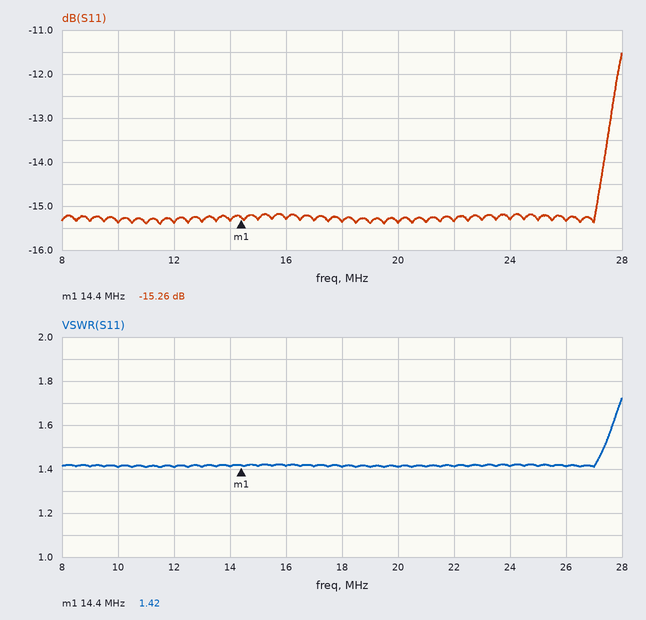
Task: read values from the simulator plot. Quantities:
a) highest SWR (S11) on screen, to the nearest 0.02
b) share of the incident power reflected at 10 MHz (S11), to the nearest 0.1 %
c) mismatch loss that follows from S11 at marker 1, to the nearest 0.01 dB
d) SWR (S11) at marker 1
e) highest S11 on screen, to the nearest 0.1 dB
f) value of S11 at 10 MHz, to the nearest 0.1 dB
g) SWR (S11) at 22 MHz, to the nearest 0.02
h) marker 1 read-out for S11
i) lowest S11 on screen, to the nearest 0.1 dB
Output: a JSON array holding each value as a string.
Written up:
["1.72", "2.9 %", "0.13 dB", "1.42", "-11.5 dB", "-15.4 dB", "1.42", "-15.26 dB", "-15.4 dB"]
